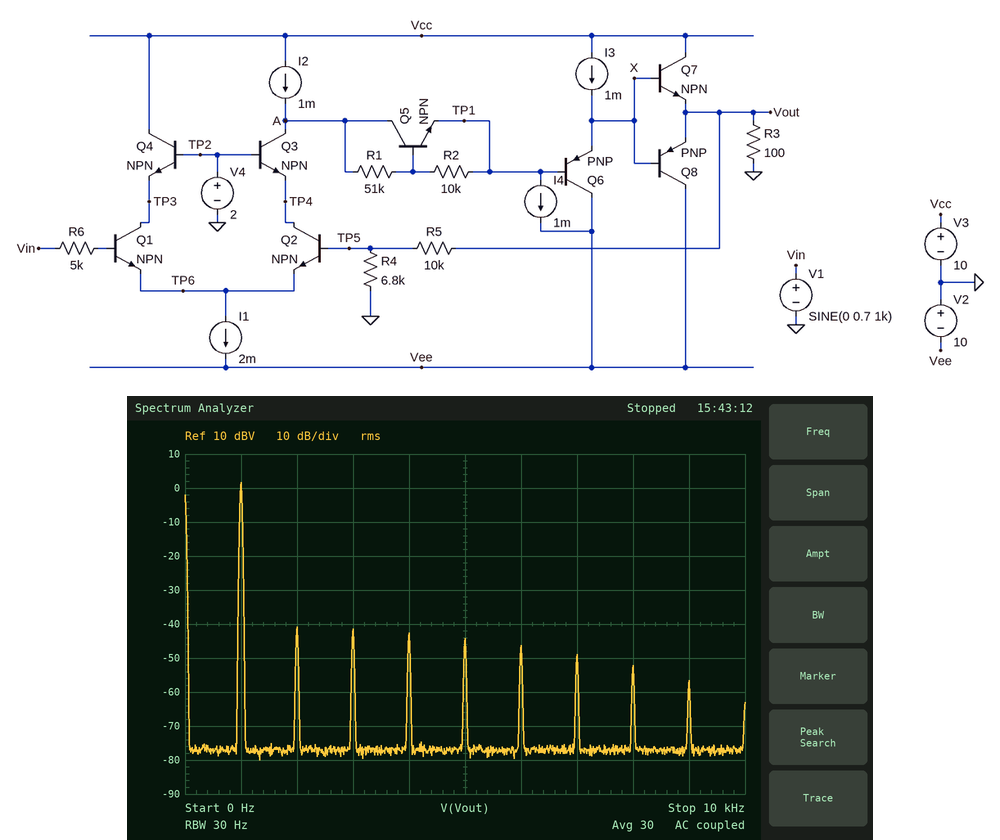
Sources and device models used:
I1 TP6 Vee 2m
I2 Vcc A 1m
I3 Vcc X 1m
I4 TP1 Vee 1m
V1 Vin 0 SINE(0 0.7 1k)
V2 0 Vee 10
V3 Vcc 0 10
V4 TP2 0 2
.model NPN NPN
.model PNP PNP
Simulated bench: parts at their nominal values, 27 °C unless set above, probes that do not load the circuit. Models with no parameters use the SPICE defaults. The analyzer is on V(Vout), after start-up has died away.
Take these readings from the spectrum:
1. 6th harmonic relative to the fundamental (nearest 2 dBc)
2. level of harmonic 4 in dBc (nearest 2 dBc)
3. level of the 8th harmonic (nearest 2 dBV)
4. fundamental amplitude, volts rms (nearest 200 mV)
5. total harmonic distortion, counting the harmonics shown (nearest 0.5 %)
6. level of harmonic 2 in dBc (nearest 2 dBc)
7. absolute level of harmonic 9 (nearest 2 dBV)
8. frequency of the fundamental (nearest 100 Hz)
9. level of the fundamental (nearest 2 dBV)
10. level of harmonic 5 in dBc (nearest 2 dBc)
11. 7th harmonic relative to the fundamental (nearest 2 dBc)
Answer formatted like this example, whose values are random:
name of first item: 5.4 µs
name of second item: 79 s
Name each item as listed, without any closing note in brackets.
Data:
6th harmonic relative to the fundamental: -48 dBc
level of harmonic 4 in dBc: -44 dBc
level of the 8th harmonic: -52 dBV
fundamental amplitude, volts rms: 1.2 V
total harmonic distortion, counting the harmonics shown: 1.5 %
level of harmonic 2 in dBc: -42 dBc
absolute level of harmonic 9: -56 dBV
frequency of the fundamental: 1.0 kHz
level of the fundamental: 2 dBV
level of harmonic 5 in dBc: -46 dBc
7th harmonic relative to the fundamental: -50 dBc
